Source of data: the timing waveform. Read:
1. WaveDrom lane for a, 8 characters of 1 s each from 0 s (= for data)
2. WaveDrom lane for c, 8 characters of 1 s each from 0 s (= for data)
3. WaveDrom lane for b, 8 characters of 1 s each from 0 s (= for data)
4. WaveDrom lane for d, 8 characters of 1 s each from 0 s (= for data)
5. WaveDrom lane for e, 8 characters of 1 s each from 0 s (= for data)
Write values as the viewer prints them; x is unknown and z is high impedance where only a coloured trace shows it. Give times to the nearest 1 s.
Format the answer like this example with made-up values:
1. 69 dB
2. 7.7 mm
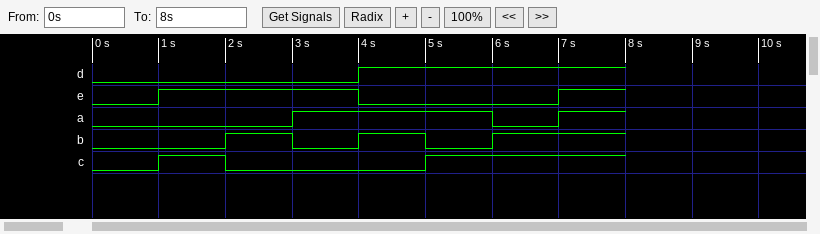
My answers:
1. {name: 'a', wave: '0..1..01'}
2. {name: 'c', wave: '010..1..'}
3. {name: 'b', wave: '0.10101.'}
4. {name: 'd', wave: '0...1...'}
5. {name: 'e', wave: '01..0..1'}
